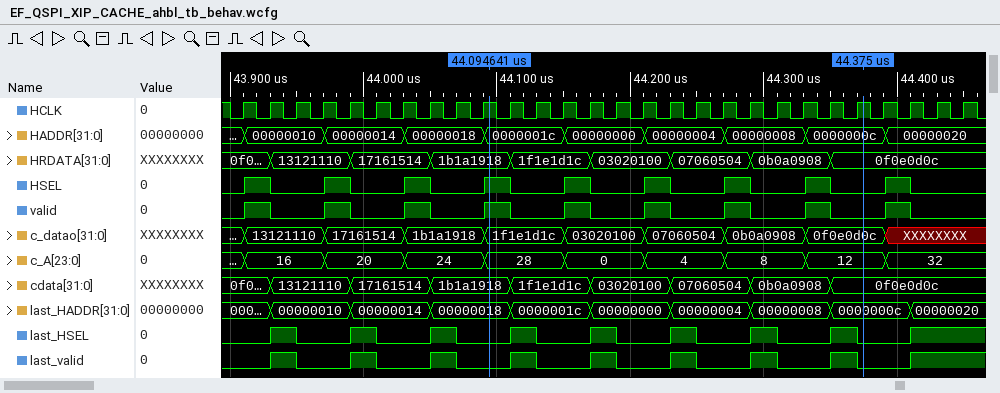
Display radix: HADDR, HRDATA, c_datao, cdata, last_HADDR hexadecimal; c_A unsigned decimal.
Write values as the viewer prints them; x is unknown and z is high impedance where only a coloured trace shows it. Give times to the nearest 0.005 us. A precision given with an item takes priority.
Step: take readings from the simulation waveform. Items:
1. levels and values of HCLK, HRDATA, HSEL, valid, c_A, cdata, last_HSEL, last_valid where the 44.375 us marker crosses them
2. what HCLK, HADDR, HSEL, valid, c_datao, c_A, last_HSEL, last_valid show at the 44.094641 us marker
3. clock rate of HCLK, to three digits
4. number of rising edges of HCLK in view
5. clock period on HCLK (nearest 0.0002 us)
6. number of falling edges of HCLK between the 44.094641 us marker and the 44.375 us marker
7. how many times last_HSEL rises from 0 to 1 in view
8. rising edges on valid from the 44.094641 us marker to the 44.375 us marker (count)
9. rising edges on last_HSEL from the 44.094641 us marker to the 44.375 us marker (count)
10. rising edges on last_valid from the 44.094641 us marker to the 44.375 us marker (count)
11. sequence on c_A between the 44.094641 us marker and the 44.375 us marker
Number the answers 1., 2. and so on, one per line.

1. HCLK=1, HRDATA=0f0e0d0c, HSEL=0, valid=0, c_A=12, cdata=0f0e0d0c, last_HSEL=0, last_valid=0
2. HCLK=1, HADDR=0000001c, HSEL=1, valid=1, c_datao=1f1e1d1c, c_A=28, last_HSEL=0, last_valid=0
3. 50.0 MHz
4. 28
5. 0.02 us
6. 14
7. 9
8. 4
9. 5
10. 5
11. 28, 0, 4, 8, 12
